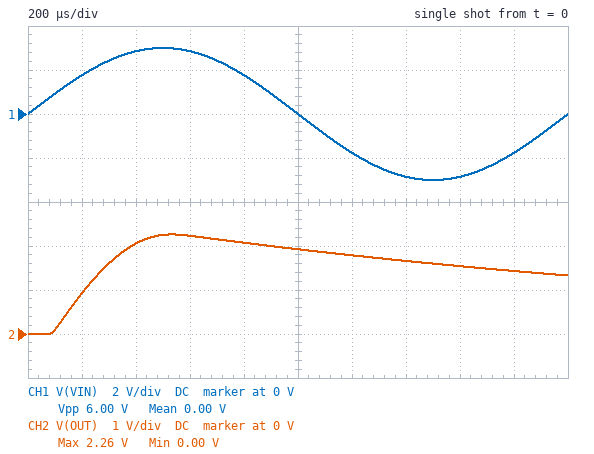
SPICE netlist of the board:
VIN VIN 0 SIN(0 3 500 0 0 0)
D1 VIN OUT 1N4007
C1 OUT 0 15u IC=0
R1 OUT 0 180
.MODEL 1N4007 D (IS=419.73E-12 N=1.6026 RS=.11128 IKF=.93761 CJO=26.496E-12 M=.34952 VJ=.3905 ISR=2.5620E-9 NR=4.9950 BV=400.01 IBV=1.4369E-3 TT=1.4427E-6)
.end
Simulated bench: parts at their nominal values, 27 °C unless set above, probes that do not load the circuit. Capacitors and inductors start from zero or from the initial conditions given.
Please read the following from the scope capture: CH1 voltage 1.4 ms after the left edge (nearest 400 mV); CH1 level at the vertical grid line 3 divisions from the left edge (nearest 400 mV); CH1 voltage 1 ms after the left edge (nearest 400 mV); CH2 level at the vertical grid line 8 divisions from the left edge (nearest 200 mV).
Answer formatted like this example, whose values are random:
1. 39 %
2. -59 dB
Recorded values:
1. -2.8 V
2. 2.8 V
3. 0 V
4. 1.6 V
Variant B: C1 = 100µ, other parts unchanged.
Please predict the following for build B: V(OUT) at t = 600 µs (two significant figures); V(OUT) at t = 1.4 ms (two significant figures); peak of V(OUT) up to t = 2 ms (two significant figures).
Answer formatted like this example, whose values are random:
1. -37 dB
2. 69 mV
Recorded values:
1. 2.2 V
2. 2.1 V
3. 2.2 V
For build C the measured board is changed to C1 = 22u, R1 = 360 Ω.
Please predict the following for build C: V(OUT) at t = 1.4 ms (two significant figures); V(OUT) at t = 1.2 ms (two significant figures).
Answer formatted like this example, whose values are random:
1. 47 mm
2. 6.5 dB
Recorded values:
1. 2.0 V
2. 2.1 V
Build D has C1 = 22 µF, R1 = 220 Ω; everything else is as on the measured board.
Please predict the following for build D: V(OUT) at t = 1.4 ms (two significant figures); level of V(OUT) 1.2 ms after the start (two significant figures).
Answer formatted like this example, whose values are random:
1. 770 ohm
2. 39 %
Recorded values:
1. 1.9 V
2. 2.0 V
